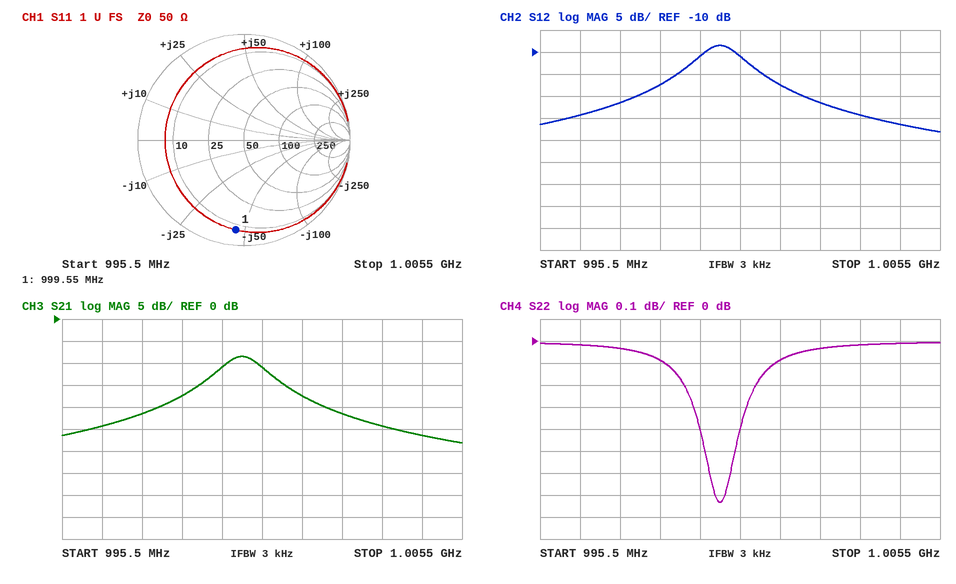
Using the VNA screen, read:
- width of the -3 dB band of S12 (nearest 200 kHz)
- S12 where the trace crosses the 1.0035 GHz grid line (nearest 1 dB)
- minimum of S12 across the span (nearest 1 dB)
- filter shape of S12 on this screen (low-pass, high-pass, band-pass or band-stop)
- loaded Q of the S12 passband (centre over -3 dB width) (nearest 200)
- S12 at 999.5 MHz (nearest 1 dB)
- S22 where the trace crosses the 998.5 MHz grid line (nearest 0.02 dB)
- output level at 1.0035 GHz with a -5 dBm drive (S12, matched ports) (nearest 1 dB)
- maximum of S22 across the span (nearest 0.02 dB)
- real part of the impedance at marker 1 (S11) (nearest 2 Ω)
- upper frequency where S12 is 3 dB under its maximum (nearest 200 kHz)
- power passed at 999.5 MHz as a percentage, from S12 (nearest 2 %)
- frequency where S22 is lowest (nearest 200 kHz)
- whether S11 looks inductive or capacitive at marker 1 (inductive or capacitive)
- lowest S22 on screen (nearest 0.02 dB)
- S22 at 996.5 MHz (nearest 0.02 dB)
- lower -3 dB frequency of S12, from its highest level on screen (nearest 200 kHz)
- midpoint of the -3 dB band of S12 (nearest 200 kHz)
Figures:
1.2 MHz
-24 dB
-28 dB
band-pass
800
-11 dB
-0.08 dB
-29 dBm
0.00 dB
8 Ω
1.0006 GHz
8 %
1.0000 GHz
capacitive
-0.74 dB
-0.02 dB
999.4 MHz
1.0000 GHz
